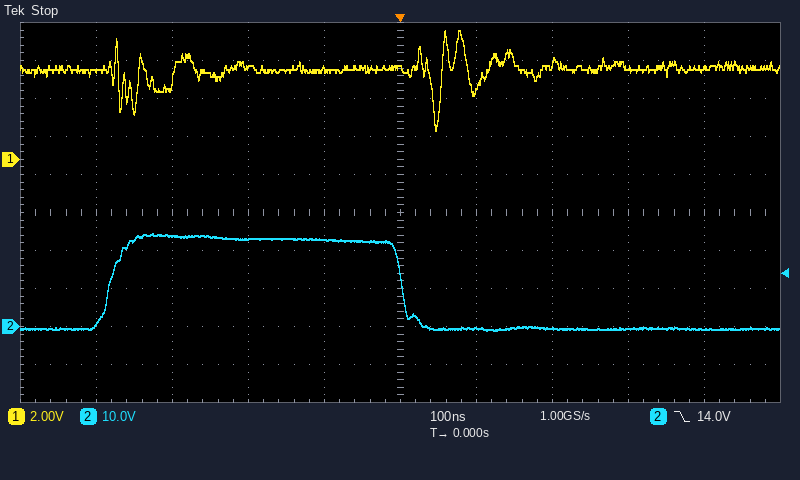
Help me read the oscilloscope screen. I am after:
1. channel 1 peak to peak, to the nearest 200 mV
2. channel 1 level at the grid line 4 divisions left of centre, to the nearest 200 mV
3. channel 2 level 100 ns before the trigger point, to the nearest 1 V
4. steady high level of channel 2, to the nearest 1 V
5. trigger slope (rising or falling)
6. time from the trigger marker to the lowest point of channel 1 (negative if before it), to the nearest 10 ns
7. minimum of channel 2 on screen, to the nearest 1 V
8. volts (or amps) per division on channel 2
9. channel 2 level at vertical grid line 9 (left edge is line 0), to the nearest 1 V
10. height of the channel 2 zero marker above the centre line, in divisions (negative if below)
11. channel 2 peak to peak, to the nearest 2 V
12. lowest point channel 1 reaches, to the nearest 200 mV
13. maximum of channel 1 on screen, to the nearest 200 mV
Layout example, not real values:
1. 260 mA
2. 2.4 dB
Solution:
1. 5.2 V
2. 4.6 V
3. 23 V
4. 23 V
5. falling
6. +50 ns
7. -1 V
8. 10 V
9. -1 V
10. -3.0 div
11. 26 V
12. 1.6 V
13. 6.8 V
